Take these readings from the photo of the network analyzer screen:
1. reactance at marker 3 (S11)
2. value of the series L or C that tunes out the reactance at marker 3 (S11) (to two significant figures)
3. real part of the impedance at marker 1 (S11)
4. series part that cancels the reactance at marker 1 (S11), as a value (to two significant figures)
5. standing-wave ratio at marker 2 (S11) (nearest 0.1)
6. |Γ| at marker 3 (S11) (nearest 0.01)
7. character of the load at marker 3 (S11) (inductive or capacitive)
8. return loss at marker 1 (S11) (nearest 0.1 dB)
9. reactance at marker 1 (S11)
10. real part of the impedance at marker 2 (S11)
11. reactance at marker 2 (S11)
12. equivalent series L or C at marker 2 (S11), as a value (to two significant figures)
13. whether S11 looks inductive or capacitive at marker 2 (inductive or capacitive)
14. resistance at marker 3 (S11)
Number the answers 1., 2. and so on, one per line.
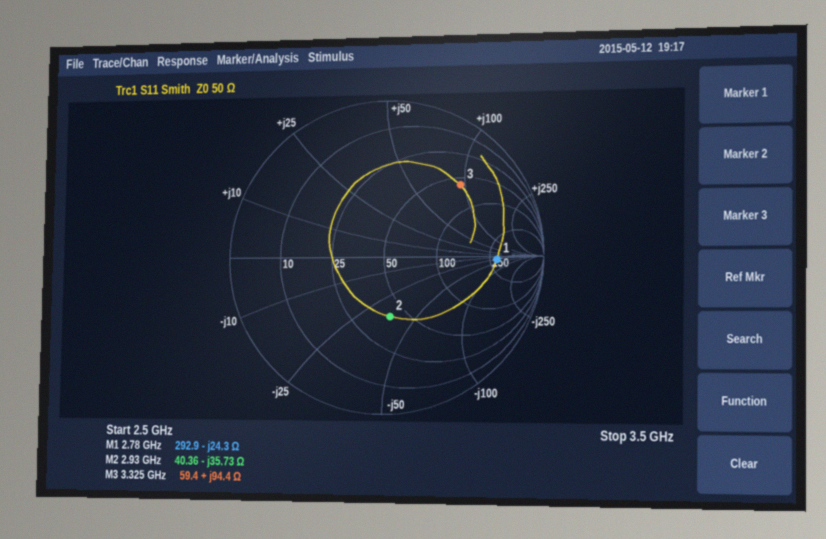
1. +94.4 Ω
2. 510 fF
3. 292.9 Ω
4. 1.4 nH
5. 2.2
6. 0.66
7. inductive
8. 3.0 dB
9. -24.3 Ω
10. 40.36 Ω
11. -35.73 Ω
12. 1.5 pF
13. capacitive
14. 59.4 Ω
